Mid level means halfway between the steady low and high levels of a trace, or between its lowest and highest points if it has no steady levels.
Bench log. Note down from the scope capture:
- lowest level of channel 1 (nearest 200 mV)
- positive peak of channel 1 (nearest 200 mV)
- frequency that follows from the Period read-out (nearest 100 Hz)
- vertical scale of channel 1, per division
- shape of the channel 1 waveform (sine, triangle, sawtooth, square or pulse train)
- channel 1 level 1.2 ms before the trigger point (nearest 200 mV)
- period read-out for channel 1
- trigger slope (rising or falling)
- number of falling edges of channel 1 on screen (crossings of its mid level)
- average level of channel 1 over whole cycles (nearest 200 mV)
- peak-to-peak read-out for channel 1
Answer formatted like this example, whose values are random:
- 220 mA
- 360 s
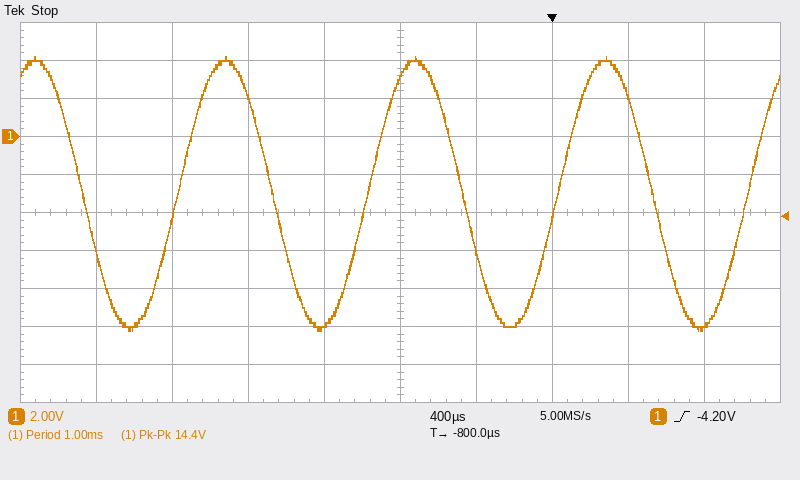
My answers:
- -10.2 V
- 4.2 V
- 1.0 kHz
- 2 V
- sine
- -10.0 V
- 1.00 ms
- rising
- 4
- -3.0 V
- 14.4 V
